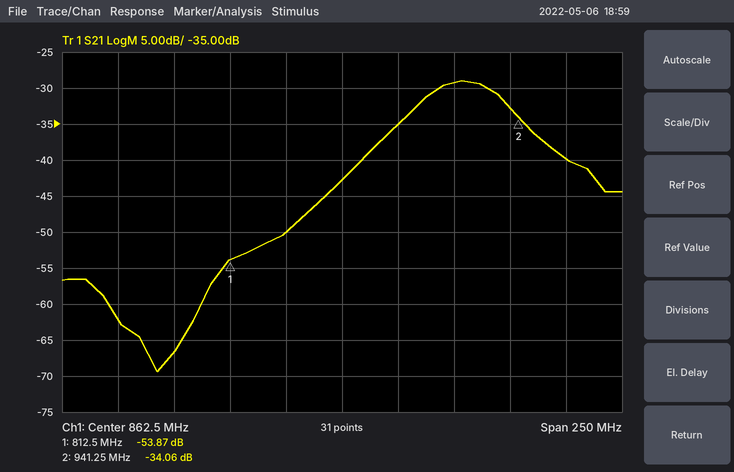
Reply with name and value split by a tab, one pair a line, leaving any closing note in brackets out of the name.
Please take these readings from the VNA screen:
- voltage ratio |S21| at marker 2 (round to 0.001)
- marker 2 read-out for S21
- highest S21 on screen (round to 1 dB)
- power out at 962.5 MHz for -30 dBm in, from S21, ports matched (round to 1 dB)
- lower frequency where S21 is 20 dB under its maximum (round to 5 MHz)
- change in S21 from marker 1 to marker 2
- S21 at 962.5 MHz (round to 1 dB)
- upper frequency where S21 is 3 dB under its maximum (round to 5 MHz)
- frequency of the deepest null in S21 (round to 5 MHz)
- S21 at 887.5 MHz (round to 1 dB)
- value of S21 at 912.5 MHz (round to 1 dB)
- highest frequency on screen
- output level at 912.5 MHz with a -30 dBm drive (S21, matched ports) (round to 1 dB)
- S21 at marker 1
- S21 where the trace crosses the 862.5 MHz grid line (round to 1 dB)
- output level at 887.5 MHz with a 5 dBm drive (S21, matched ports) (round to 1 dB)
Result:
voltage ratio |S21| at marker 2	0.020
marker 2 read-out for S21	-34.06 dB
highest S21 on screen	-29 dB
power out at 962.5 MHz for -30 dBm in, from S21, ports matched	-70 dBm
lower frequency where S21 is 20 dB under its maximum	840 MHz
change in S21 from marker 1 to marker 2	19.81 dB
S21 at 962.5 MHz	-40 dB
upper frequency where S21 is 3 dB under its maximum	935 MHz
frequency of the deepest null in S21	780 MHz
S21 at 887.5 MHz	-35 dB
value of S21 at 912.5 MHz	-29 dB
highest frequency on screen	987.5 MHz
output level at 912.5 MHz with a -30 dBm drive (S21, matched ports)	-59 dBm
S21 at marker 1	-53.87 dB
S21 where the trace crosses the 862.5 MHz grid line	-43 dB
output level at 887.5 MHz with a 5 dBm drive (S21, matched ports)	-30 dBm
